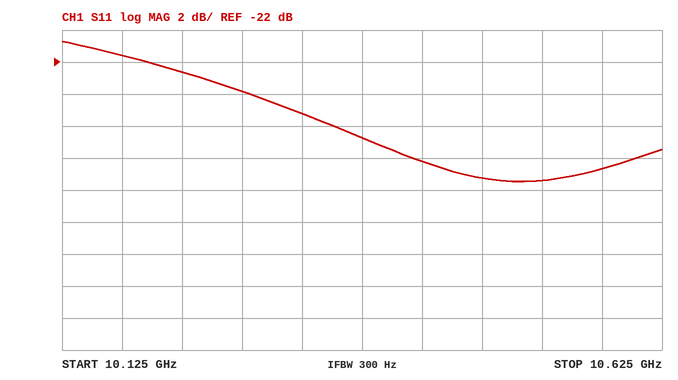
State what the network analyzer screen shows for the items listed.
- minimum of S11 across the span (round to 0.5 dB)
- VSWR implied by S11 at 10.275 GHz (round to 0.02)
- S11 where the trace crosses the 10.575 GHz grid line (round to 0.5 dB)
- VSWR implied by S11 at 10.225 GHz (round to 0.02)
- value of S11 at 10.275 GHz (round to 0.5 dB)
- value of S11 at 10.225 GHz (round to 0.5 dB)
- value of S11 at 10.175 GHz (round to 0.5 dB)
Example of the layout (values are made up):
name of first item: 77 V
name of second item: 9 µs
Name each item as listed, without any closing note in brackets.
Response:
minimum of S11 across the span: -29.5 dB
VSWR implied by S11 at 10.275 GHz: 1.14
S11 where the trace crosses the 10.575 GHz grid line: -28.5 dB
VSWR implied by S11 at 10.225 GHz: 1.16
value of S11 at 10.275 GHz: -24.0 dB
value of S11 at 10.225 GHz: -22.5 dB
value of S11 at 10.175 GHz: -21.5 dB
